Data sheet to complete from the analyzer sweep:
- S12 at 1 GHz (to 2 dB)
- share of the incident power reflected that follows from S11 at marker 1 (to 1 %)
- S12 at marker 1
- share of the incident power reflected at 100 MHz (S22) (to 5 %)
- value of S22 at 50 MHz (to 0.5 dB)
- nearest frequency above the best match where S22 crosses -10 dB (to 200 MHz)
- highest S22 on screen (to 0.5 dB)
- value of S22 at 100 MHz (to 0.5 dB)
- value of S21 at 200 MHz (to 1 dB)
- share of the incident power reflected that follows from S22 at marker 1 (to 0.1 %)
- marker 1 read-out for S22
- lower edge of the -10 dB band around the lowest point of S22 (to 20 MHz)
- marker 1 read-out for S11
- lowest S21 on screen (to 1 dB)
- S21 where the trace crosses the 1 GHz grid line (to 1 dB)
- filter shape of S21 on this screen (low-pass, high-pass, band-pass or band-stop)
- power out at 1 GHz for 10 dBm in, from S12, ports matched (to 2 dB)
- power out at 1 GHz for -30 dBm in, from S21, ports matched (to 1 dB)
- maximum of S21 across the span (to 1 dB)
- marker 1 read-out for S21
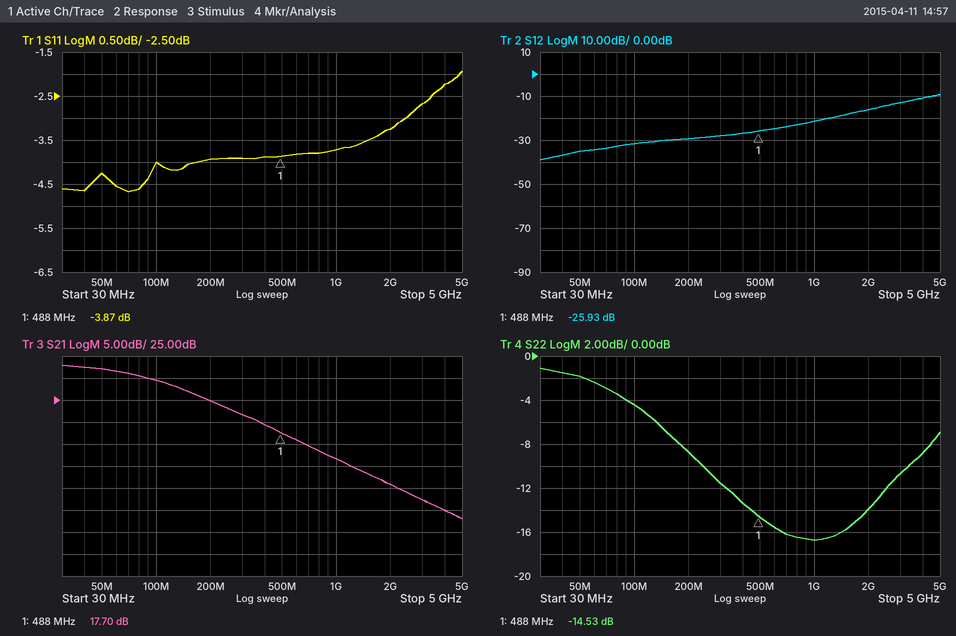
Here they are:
-22 dB
41 %
-25.93 dB
35 %
-2.0 dB
3.4 GHz
-1.0 dB
-4.5 dB
25 dB
3.5 %
-14.53 dB
240 MHz
-3.87 dB
-2 dB
12 dB
low-pass
-12 dBm
-18 dBm
33 dB
17.70 dB
